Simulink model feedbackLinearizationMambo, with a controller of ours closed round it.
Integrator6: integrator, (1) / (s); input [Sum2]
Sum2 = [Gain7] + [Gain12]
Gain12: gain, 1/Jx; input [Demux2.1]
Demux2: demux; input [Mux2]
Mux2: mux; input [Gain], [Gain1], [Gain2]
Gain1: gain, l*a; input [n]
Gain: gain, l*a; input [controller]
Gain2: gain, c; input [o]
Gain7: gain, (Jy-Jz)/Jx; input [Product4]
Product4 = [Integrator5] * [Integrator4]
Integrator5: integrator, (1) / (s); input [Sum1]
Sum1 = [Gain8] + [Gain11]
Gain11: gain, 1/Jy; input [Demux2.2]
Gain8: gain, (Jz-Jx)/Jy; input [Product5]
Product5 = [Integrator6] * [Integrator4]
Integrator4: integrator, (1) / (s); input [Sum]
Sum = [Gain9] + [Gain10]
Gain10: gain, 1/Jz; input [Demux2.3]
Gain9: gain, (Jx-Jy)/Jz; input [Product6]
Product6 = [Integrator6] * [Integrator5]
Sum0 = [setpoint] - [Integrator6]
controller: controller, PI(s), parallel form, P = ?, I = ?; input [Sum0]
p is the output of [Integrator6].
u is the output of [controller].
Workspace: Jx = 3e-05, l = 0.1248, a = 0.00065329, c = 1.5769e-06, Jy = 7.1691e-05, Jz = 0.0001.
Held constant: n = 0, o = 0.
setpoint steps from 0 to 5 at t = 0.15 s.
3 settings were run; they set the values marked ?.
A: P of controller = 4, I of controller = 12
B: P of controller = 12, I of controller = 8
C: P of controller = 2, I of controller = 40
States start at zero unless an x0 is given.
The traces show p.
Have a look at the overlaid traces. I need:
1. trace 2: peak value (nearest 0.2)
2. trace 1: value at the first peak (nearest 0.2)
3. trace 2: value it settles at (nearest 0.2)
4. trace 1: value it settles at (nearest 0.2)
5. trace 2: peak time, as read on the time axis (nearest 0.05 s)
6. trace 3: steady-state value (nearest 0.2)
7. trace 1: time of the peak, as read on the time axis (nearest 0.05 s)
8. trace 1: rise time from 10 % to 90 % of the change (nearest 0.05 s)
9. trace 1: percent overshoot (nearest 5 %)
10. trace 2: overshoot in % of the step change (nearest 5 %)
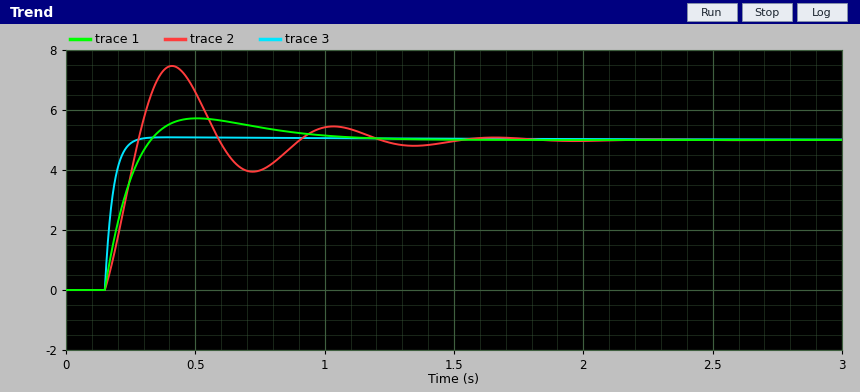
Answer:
7.4
5.8
5.0
5.0
0.40 s
5.0
0.50 s
0.15 s
15 %
50 %
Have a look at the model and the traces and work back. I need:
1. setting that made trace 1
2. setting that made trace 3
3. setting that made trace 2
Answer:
A
B
C
